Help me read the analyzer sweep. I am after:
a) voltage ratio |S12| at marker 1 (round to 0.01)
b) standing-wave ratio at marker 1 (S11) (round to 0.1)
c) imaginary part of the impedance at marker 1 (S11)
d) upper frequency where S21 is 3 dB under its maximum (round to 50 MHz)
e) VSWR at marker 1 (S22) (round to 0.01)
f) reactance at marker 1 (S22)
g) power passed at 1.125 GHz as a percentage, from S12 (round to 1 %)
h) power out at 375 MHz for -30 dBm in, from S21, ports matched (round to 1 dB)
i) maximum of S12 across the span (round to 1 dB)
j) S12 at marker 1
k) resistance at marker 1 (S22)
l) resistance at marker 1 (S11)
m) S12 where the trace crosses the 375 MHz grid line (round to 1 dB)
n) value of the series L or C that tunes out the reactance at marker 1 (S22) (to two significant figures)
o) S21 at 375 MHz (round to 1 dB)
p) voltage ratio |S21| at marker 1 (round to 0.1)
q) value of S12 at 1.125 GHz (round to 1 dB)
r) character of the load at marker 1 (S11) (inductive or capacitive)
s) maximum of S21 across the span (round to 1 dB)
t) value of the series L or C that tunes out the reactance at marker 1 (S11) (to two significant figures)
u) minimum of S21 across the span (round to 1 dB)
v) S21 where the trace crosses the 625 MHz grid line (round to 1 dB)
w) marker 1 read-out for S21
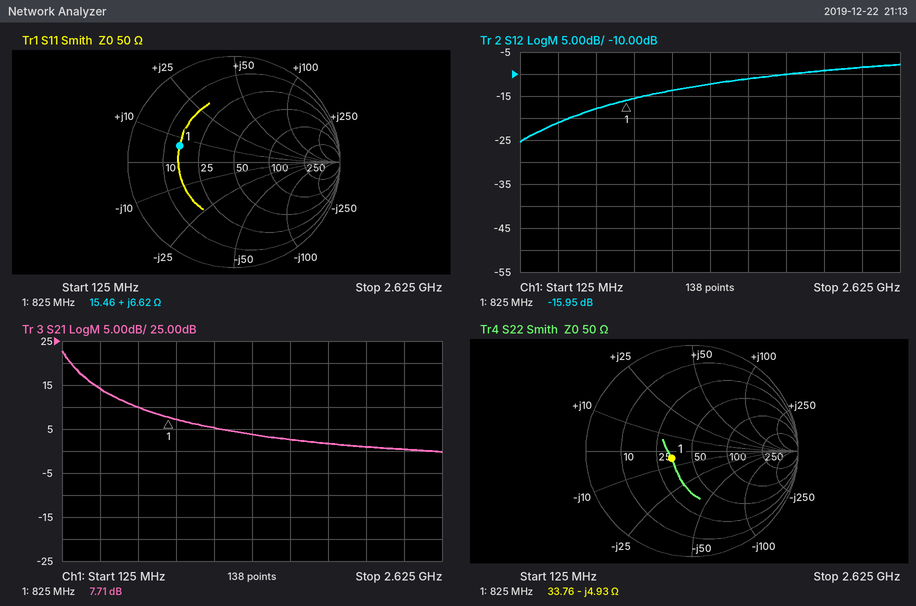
0.16
3.3
+6.62 Ω
200 MHz
1.51
-4.93 Ω
4 %
-16 dBm
-8 dB
-15.95 dB
33.76 Ω
15.46 Ω
-21 dB
950 pH
14 dB
2.4
-14 dB
inductive
23 dB
29 pF
0 dB
10 dB
7.71 dB
